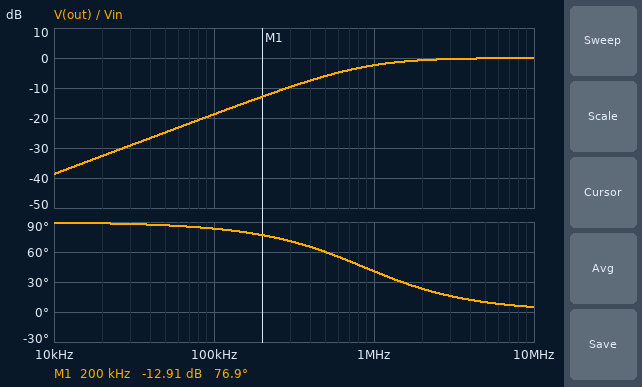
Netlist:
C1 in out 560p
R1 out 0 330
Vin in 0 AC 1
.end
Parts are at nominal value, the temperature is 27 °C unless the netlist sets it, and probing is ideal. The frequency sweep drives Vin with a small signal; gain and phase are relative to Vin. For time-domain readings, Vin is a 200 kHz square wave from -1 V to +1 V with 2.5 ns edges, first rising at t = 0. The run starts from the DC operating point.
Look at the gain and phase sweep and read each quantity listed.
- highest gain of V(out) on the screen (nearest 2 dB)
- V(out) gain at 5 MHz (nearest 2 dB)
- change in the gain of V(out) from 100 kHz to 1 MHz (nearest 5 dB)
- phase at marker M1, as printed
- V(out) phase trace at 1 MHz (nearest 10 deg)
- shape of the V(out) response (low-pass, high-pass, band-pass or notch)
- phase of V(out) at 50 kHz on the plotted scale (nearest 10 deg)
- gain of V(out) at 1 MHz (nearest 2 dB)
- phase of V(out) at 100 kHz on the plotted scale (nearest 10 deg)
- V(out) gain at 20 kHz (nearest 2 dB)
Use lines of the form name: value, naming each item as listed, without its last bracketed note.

highest gain of V(out) on the screen: 0 dB
V(out) gain at 5 MHz: 0 dB
change in the gain of V(out) from 100 kHz to 1 MHz: 15 dB
phase at marker M1, as printed: 76.9 deg
V(out) phase trace at 1 MHz: 40 deg
shape of the V(out) response: high-pass
phase of V(out) at 50 kHz on the plotted scale: 90 deg
gain of V(out) at 1 MHz: -2 dB
phase of V(out) at 100 kHz on the plotted scale: 80 deg
V(out) gain at 20 kHz: -32 dB
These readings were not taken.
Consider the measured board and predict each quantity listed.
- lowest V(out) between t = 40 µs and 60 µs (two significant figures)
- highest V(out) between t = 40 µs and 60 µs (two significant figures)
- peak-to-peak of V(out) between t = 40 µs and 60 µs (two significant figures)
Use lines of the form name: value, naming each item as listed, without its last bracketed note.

lowest V(out) between t = 40 µs and 60 µs: -2.0 V
highest V(out) between t = 40 µs and 60 µs: 2.0 V
peak-to-peak of V(out) between t = 40 µs and 60 µs: 4.0 V
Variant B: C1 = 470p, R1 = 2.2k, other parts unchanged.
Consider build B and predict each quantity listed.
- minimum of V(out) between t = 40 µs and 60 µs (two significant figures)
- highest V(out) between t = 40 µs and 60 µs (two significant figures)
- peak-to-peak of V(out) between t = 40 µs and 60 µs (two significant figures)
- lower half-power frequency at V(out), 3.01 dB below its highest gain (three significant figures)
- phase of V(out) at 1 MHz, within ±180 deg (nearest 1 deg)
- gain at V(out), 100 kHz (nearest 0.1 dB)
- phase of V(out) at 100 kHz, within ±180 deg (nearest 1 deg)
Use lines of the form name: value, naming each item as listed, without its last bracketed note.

minimum of V(out) between t = 40 µs and 60 µs: -1.8 V
highest V(out) between t = 40 µs and 60 µs: 1.8 V
peak-to-peak of V(out) between t = 40 µs and 60 µs: 3.7 V
lower half-power frequency at V(out), 3.01 dB below its highest gain: 154 kHz
phase of V(out) at 1 MHz, within ±180 deg: 9 deg
gain at V(out), 100 kHz: -5.3 dB
phase of V(out) at 100 kHz, within ±180 deg: 57 deg
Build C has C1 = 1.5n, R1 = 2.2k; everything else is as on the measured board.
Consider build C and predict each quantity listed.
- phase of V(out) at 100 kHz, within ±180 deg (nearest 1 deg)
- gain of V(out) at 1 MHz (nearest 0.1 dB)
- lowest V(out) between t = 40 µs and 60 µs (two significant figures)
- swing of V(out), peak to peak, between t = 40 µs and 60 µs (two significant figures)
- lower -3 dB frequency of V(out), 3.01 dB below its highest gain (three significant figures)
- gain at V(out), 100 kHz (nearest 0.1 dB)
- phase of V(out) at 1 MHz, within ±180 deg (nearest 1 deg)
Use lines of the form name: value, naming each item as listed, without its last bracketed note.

phase of V(out) at 100 kHz, within ±180 deg: 26 deg
gain of V(out) at 1 MHz: 0 dB
lowest V(out) between t = 40 µs and 60 µs: -1.4 V
swing of V(out), peak to peak, between t = 40 µs and 60 µs: 2.7 V
lower -3 dB frequency of V(out), 3.01 dB below its highest gain: 48.2 kHz
gain at V(out), 100 kHz: -0.9 dB
phase of V(out) at 1 MHz, within ±180 deg: 3 deg
